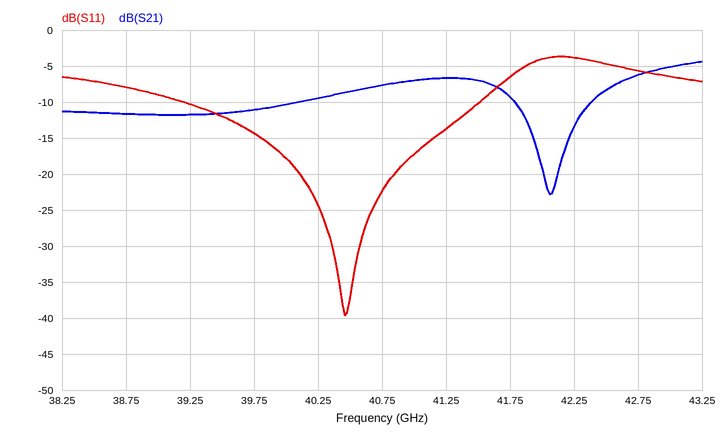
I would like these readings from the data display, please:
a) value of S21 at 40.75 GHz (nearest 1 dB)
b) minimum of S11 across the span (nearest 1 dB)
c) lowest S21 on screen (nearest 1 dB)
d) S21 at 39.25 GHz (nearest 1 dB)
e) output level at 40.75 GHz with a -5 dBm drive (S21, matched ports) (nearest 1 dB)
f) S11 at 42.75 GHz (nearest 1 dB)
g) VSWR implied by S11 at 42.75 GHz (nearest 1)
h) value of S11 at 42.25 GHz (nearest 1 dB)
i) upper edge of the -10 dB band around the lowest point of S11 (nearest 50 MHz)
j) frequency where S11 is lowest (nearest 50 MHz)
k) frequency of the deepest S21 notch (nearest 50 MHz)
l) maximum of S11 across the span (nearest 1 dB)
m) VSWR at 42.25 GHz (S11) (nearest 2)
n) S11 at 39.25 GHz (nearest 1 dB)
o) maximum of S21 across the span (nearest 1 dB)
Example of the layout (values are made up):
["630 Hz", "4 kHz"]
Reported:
["-8 dB", "-40 dB", "-23 dB", "-12 dB", "-13 dBm", "-6 dB", "3", "-4 dB", "41.50 GHz", "40.45 GHz", "42.05 GHz", "-4 dB", "4", "-10 dB", "-4 dB"]
